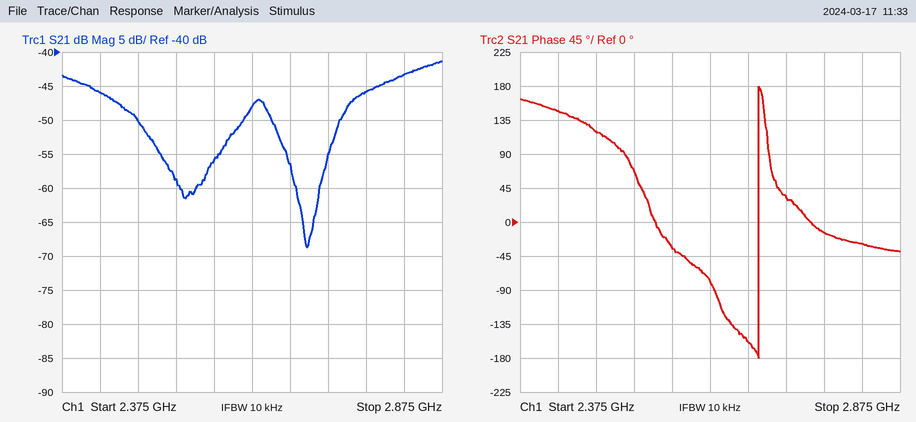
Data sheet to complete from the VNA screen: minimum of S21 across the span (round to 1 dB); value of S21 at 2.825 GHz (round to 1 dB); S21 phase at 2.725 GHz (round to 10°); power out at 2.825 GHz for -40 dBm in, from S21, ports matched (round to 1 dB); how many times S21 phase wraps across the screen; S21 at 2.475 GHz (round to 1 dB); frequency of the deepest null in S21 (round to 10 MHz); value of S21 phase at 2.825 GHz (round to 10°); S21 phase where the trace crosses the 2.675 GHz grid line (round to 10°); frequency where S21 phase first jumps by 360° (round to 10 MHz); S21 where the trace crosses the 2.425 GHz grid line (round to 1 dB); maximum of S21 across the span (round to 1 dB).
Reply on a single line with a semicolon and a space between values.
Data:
-69 dB; -43 dB; 30°; -83 dBm; 1; -50 dB; 2.70 GHz; -30°; -160°; 2.69 GHz; -46 dB; -41 dB
